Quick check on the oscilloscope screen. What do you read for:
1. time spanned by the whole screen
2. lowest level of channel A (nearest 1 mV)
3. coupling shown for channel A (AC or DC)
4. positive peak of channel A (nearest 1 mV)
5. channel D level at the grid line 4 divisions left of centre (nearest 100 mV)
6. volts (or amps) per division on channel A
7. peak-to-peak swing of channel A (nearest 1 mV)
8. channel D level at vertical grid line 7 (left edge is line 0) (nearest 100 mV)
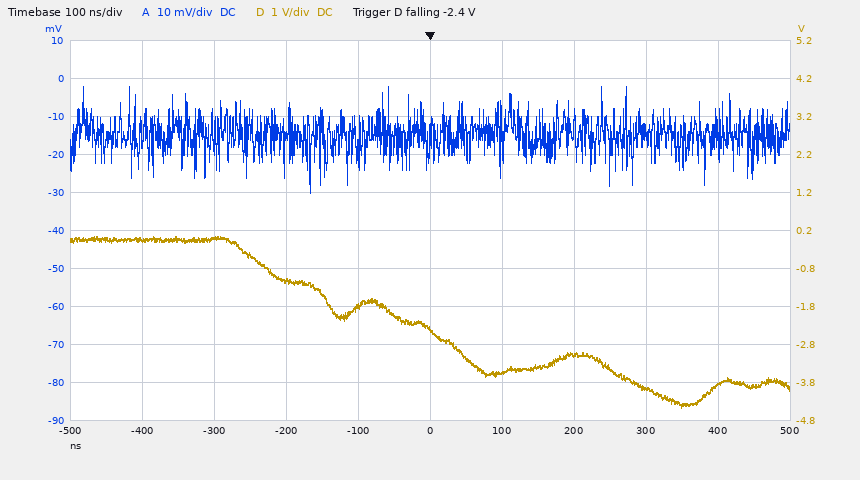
1 µs
-30 mV
DC
-2 mV
0.0 V
10 mV
28 mV
-3.1 V
